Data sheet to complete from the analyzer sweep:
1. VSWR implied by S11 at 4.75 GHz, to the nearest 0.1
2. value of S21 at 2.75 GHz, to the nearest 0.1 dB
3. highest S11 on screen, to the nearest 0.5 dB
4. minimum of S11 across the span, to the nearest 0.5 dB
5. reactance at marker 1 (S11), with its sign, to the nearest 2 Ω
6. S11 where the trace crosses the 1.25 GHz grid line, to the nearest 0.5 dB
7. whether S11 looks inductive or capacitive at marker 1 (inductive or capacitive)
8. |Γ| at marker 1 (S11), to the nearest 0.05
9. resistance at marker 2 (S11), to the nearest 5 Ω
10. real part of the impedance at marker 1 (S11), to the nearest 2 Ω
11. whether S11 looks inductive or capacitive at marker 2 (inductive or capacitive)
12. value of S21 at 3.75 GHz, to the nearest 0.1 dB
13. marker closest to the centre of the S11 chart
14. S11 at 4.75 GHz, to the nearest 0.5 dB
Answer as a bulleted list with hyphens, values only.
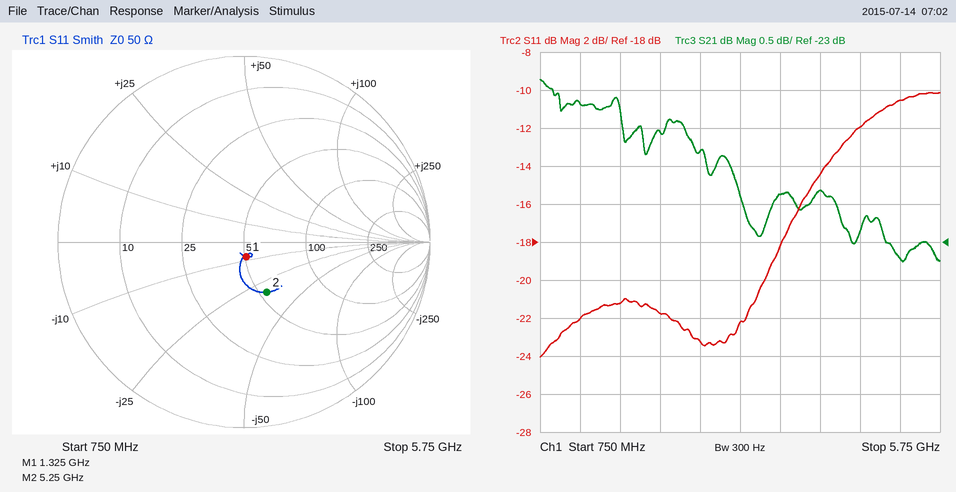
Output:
- 1.7
- -21.8 dB
- -10.0 dB
- -24.0 dB
- -8 Ω
- -22.0 dB
- capacitive
- 0.10
- 55 Ω
- 50 Ω
- capacitive
- -22.4 dB
- marker 1
- -12.0 dB
